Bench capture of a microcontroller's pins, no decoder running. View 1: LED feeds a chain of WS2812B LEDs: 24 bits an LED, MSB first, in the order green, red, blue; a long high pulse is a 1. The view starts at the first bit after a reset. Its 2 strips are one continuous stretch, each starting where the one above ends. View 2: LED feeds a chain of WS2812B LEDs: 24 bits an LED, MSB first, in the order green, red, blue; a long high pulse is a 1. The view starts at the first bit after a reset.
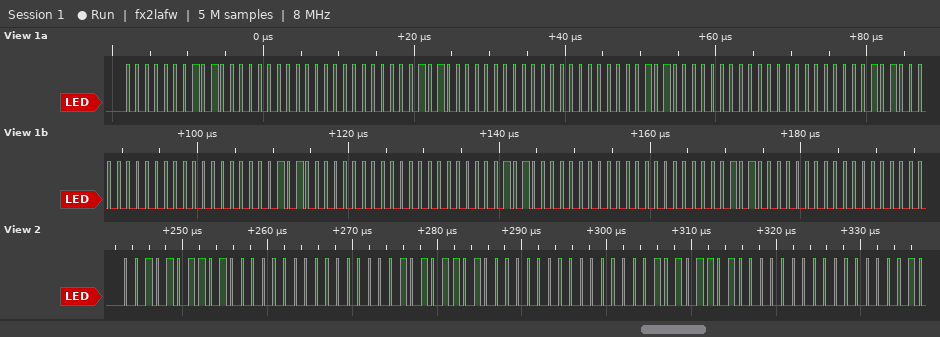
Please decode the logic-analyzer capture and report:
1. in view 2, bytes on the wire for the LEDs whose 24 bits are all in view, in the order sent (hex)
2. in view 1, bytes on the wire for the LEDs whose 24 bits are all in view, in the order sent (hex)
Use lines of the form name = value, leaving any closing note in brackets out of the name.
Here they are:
in view 2, bytes on the wire for the LEDs whose 24 bits are all in view, in the order sent = 2B 40 00 2B 40 00 2B 40 00
in view 1, bytes on the wire for the LEDs whose 24 bits are all in view, in the order sent = 01 40 00 01 40 00 01 40 00 01 40 00 01 40 00 01 40 00 01 40 00
